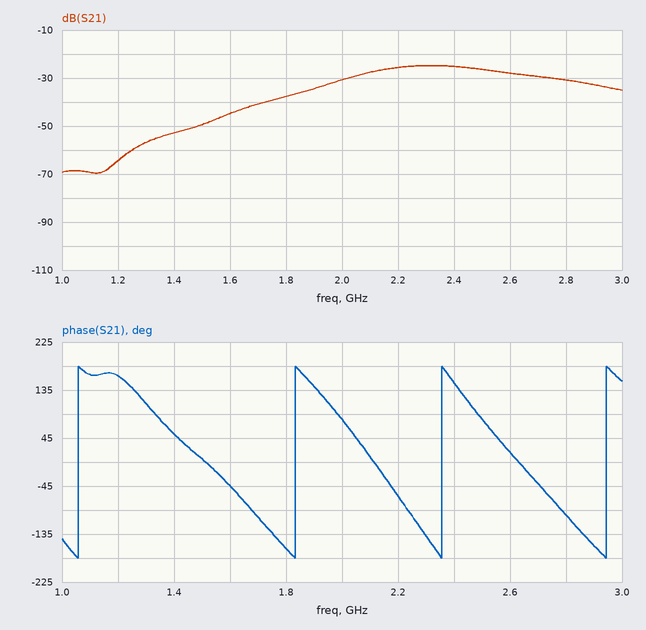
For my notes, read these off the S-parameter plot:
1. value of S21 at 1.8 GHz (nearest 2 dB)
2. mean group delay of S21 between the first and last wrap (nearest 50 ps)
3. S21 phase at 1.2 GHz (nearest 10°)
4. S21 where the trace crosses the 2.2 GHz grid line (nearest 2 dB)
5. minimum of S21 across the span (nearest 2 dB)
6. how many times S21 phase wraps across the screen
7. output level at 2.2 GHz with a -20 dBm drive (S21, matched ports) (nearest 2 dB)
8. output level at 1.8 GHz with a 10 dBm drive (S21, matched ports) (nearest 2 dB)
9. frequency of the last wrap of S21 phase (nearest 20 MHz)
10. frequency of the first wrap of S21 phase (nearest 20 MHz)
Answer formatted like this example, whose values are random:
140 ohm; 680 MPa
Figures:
-38 dB; 1.60 ns; 160°; -26 dB; -70 dB; 4; -46 dBm; -28 dBm; 2.94 GHz; 1.06 GHz
